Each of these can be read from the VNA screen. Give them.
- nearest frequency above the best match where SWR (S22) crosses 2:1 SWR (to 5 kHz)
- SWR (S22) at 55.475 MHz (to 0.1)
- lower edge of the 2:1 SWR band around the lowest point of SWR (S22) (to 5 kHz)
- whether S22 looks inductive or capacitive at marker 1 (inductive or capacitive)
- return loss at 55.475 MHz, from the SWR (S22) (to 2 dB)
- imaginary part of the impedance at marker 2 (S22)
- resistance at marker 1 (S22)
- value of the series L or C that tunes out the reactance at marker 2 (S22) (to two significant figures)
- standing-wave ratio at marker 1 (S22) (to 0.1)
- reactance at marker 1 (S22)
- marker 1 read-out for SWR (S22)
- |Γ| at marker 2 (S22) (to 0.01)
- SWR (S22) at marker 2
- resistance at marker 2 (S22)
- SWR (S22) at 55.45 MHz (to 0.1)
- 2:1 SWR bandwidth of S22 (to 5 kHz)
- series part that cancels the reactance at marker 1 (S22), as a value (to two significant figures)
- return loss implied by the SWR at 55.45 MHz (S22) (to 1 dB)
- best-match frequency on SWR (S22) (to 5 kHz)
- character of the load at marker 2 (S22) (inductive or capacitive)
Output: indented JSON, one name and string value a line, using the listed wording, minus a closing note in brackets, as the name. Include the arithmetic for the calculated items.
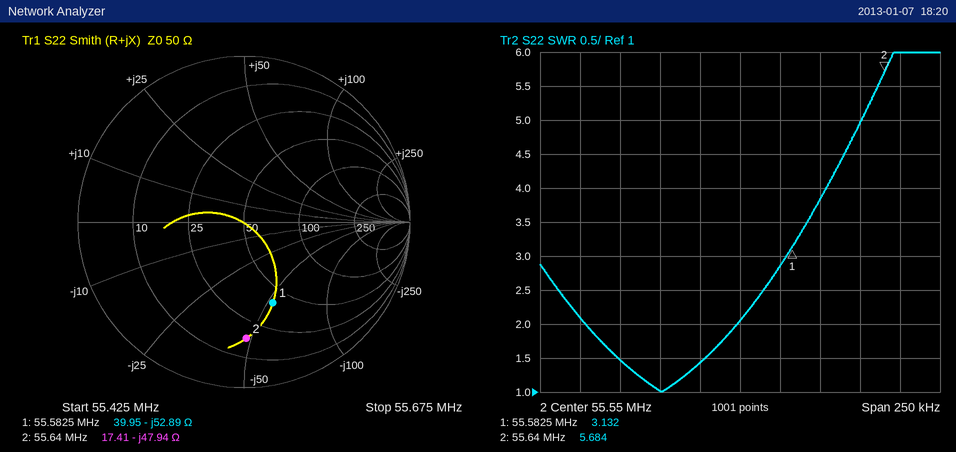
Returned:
{
  "nearest frequency above the best match where SWR (S22) crosses 2:1 SWR": "55.550 MHz",
  "SWR (S22) at 55.475 MHz": "1.5",
  "lower edge of the 2:1 SWR band around the lowest point of SWR (S22)": "55.455 MHz",
  "whether S22 looks inductive or capacitive at marker 1": "capacitive",
  "return loss at 55.475 MHz, from the SWR (S22)": "−20 log10((1.5 − 1)/(1.5 + 1)) ≈ 14 dB",
  "imaginary part of the impedance at marker 2": "-47.94 Ω",
  "resistance at marker 1": "39.95 Ω",
  "value of the series L or C that tunes out the reactance at marker 2 (S22)": "L = 47.94 Ω/(2π × 55.64 MHz) ≈ 137 nH, so 140 nH to two significant figures",
  "standing-wave ratio at marker 1 (S22)": "3.1",
  "reactance at marker 1": "-52.89 Ω",
  "marker 1 read-out for SWR": "3.132",
  "|Γ| at marker 2 (S22)": "0.70",
  "SWR (S22) at marker 2": "5.684",
  "resistance at marker 2": "17.41 Ω",
  "SWR (S22) at 55.45 MHz": "2.1",
  "2:1 SWR bandwidth of S22": "55.550 MHz − 55.455 MHz = 95 kHz",
  "series part that cancels the reactance at marker 1 (S22), as a value": "L = 52.89 Ω/(2π × 55.5825 MHz) ≈ 151 nH, so 150 nH to two significant figures",
  "return loss implied by the SWR at 55.45 MHz (S22)": "−20 log10((2.1 − 1)/(2.1 + 1)) ≈ 9 dB",
  "best-match frequency on SWR (S22)": "55.500 MHz",
  "character of the load at marker 2 (S22)": "capacitive"
}
